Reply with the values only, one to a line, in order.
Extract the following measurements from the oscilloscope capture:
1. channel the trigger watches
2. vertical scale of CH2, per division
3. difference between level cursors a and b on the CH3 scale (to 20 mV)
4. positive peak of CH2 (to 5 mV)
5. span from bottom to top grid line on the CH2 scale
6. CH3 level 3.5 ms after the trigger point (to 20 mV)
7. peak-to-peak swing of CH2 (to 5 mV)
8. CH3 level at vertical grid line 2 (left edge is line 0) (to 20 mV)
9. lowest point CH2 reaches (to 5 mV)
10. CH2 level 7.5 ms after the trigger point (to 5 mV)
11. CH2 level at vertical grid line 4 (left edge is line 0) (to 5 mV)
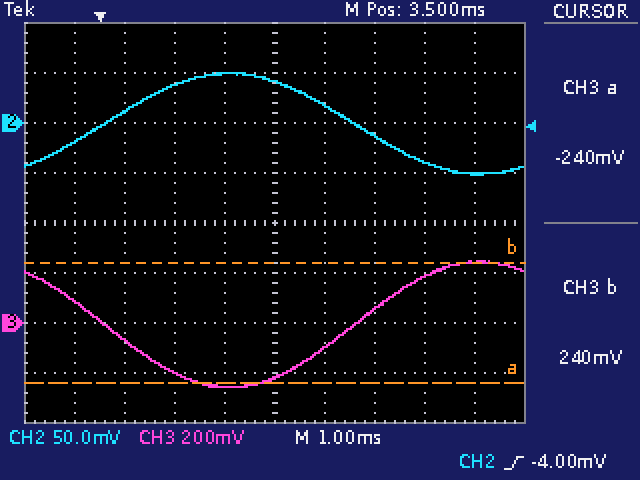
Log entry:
CH2
50 mV
480 mV
50 mV
400 mV
-220 mV
100 mV
-60 mV
-50 mV
-50 mV
50 mV
